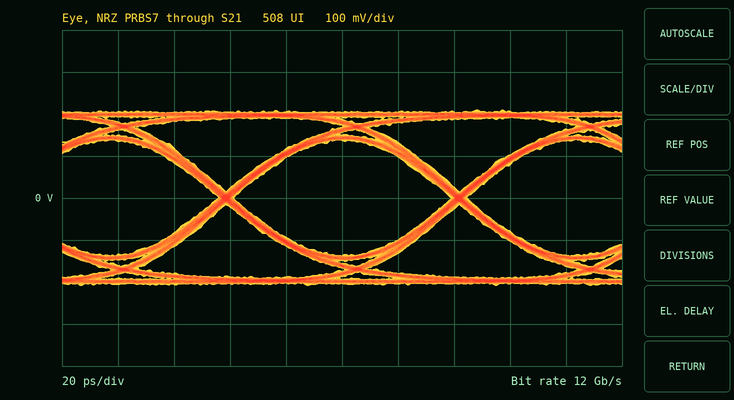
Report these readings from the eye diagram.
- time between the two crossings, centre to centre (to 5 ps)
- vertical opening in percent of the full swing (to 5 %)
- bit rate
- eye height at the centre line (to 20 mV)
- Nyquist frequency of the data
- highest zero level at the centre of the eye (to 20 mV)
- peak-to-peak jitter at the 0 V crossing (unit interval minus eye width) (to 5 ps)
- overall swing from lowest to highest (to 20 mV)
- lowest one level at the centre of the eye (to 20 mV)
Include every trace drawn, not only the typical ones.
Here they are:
85 ps
65 %
12 Gb/s
280 mV
6 GHz
-140 mV
5 ps
420 mV
140 mV
